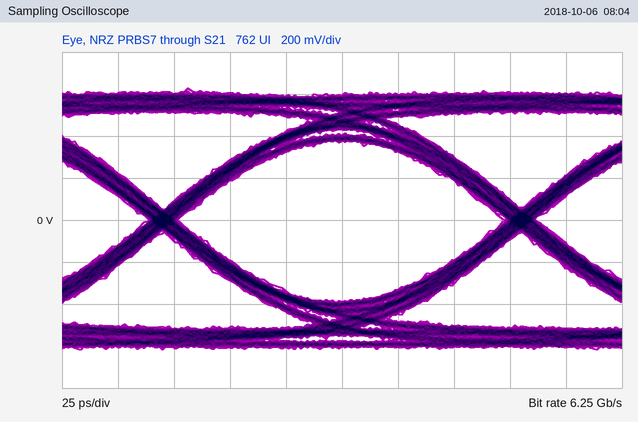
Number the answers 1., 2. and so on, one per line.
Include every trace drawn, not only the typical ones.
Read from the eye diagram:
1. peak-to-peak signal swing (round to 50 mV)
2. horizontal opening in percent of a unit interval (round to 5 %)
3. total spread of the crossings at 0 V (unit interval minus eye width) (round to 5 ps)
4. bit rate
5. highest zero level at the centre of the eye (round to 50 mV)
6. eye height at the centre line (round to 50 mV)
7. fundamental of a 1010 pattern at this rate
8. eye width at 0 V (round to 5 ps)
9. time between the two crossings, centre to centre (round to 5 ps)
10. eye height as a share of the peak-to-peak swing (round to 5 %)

1. 1.25 V
2. 90 %
3. 15 ps
4. 6.25 Gb/s
5. -400 mV
6. 750 mV
7. 3.125 GHz
8. 145 ps
9. 160 ps
10. 60 %
